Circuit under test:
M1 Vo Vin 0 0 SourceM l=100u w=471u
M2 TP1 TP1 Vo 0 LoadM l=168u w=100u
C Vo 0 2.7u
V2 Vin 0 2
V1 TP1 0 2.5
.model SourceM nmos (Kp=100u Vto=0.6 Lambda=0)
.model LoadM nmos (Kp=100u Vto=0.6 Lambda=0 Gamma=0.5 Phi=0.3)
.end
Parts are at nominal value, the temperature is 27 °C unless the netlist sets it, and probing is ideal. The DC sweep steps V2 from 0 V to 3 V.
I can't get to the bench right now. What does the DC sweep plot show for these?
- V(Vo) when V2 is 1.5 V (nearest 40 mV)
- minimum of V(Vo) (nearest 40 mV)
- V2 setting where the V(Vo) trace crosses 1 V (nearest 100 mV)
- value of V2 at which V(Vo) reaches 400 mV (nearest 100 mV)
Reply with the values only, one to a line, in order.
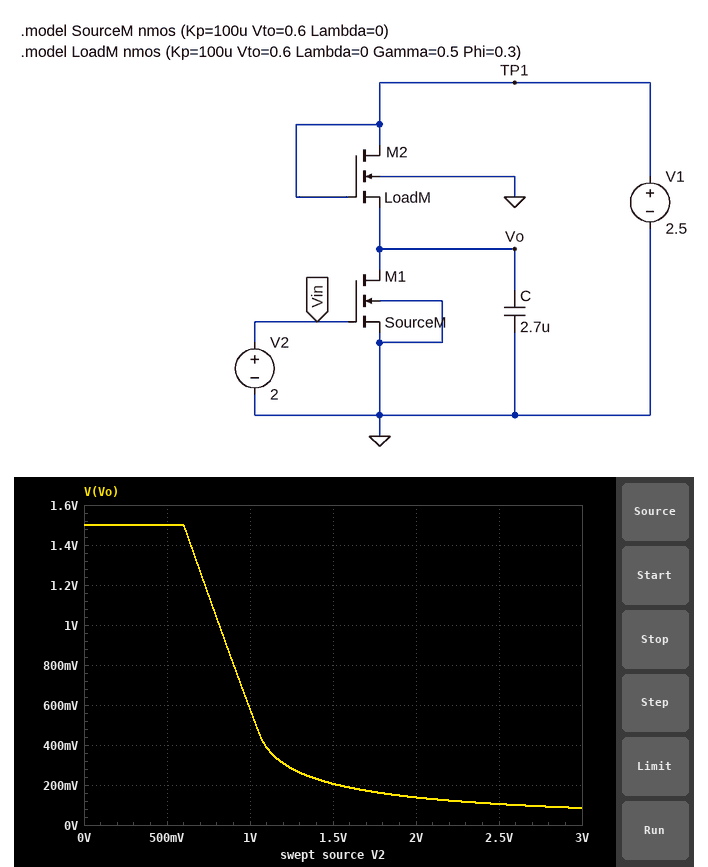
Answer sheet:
200 mV
80 mV
800 mV
1.1 V
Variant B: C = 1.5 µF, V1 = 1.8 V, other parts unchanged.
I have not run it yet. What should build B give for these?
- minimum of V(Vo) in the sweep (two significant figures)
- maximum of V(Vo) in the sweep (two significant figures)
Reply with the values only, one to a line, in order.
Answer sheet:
35 mV
920 mV
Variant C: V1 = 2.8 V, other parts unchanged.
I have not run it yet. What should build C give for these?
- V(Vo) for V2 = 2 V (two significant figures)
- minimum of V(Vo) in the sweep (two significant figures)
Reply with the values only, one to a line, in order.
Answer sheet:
180 mV
110 mV
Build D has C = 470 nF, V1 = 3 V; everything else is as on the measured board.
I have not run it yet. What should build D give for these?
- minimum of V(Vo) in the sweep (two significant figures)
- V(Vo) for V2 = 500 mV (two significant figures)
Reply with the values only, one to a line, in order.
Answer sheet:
130 mV
1.9 V
